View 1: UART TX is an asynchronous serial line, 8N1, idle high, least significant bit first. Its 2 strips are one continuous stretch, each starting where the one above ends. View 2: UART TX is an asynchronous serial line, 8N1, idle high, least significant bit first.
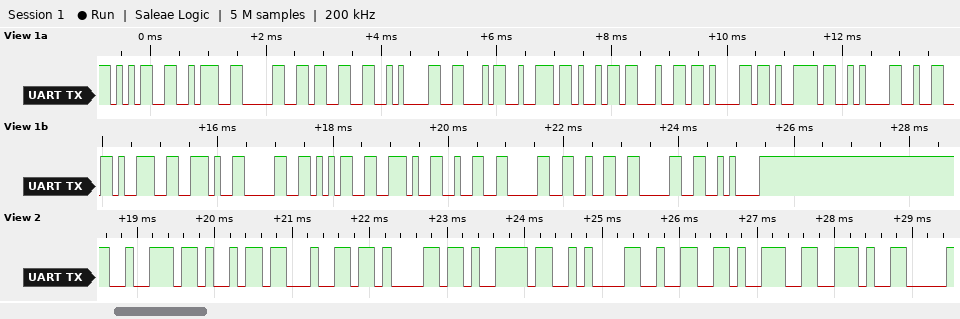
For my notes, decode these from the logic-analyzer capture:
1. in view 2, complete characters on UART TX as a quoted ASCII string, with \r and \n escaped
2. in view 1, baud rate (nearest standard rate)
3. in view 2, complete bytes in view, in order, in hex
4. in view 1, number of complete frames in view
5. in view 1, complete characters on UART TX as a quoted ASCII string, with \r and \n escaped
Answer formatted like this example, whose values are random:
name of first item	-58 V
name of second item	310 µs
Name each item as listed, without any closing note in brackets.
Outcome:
in view 2, complete characters on UART TX as a quoted ASCII string, with \r and \n escaped	"riday\n29."
in view 1, baud rate	9600 baud
in view 2, complete bytes in view, in order, in hex	0x72 0x69 0x64 0x61 0x79 0x0A 0x32 0x39 0x2E
in view 1, number of complete frames in view	23
in view 1, complete characters on UART TX as a quoted ASCII string, with \r and \n escaped	"5:03\nFriday\n29.05.2020\n"
